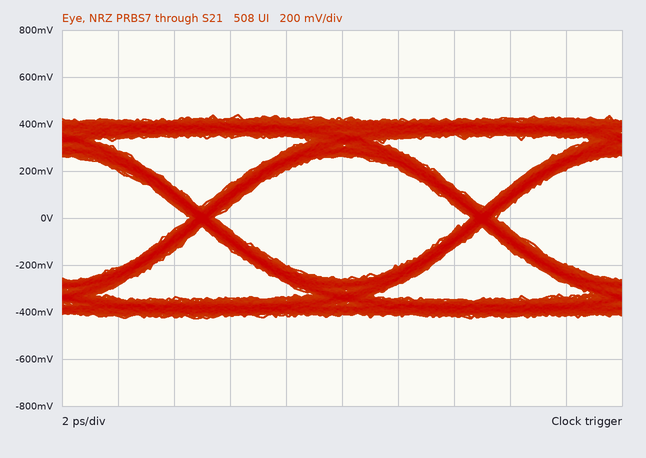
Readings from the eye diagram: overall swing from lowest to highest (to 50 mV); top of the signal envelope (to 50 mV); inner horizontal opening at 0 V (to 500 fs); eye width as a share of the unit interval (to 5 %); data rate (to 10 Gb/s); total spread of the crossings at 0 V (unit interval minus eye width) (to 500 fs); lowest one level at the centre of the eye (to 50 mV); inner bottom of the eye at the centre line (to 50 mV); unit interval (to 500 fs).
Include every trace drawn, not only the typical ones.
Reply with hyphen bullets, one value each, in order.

- 850 mV
- 450 mV
- 9.0 ps
- 90 %
- 100 Gb/s
- 1.0 ps
- 250 mV
- -250 mV
- 10.0 ps
